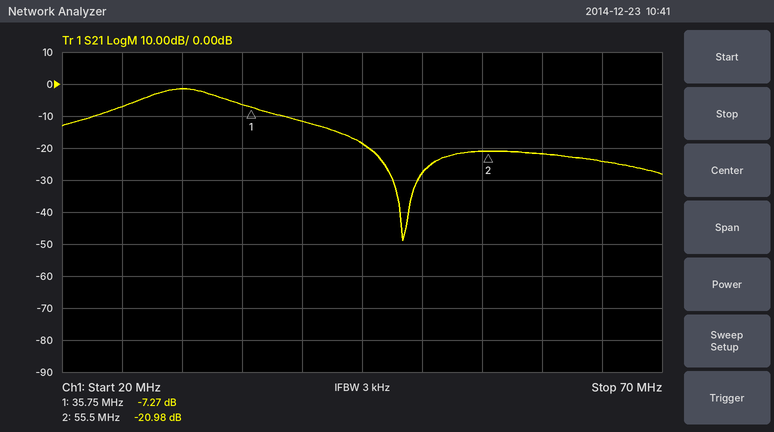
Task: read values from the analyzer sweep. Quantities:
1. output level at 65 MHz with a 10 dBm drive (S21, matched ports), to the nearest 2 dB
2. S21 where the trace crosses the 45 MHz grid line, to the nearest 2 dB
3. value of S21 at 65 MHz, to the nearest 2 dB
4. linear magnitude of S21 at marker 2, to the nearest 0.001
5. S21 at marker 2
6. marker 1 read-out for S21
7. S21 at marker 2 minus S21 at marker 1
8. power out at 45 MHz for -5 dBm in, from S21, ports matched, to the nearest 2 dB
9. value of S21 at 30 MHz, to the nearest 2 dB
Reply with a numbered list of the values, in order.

1. -14 dBm
2. -18 dB
3. -24 dB
4. 0.089
5. -20.98 dB
6. -7.27 dB
7. -13.71 dB
8. -24 dBm
9. -2 dB
